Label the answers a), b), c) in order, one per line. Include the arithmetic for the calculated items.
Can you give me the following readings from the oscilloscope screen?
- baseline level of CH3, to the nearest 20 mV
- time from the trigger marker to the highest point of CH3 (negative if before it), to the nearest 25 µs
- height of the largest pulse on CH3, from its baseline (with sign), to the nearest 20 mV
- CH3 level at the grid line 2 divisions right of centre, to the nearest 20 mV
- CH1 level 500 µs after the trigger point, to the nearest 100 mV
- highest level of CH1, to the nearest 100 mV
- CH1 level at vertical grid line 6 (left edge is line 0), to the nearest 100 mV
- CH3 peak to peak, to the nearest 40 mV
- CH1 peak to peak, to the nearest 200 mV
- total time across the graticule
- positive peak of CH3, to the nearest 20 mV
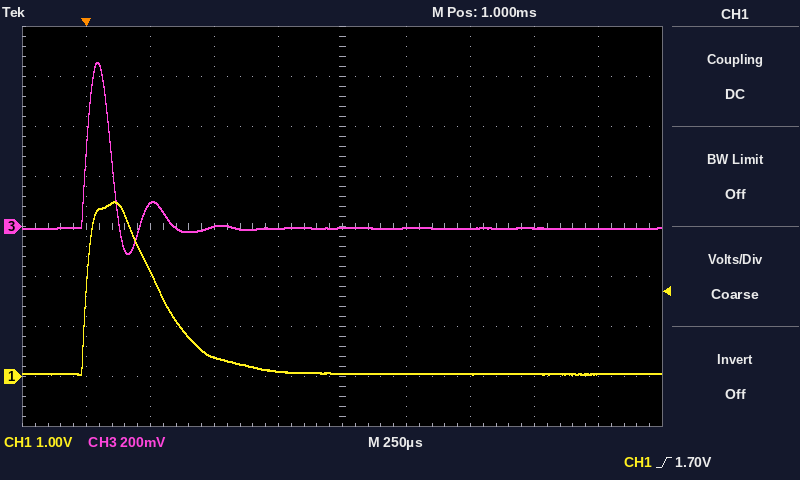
a) 0 mV
b) +50 µs
c) 660 mV − (0 mV) = +660 mV
d) 0 mV
e) 400 mV
f) 3.5 V
g) 100 mV
h) 760 mV
i) 3.4 V
j) 2.5 ms
k) 660 mV
